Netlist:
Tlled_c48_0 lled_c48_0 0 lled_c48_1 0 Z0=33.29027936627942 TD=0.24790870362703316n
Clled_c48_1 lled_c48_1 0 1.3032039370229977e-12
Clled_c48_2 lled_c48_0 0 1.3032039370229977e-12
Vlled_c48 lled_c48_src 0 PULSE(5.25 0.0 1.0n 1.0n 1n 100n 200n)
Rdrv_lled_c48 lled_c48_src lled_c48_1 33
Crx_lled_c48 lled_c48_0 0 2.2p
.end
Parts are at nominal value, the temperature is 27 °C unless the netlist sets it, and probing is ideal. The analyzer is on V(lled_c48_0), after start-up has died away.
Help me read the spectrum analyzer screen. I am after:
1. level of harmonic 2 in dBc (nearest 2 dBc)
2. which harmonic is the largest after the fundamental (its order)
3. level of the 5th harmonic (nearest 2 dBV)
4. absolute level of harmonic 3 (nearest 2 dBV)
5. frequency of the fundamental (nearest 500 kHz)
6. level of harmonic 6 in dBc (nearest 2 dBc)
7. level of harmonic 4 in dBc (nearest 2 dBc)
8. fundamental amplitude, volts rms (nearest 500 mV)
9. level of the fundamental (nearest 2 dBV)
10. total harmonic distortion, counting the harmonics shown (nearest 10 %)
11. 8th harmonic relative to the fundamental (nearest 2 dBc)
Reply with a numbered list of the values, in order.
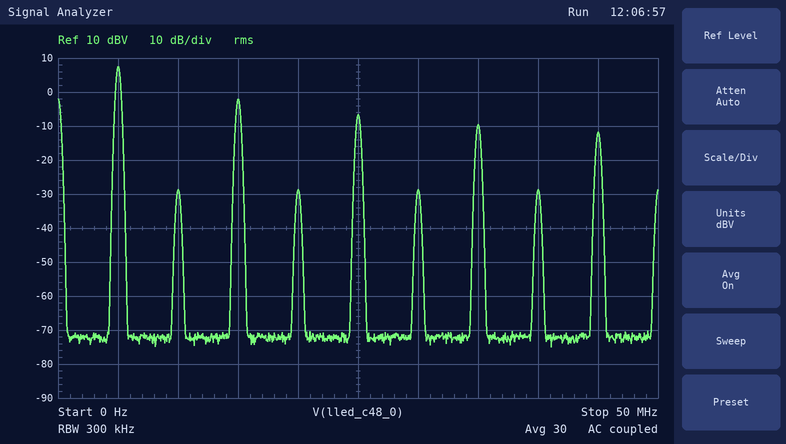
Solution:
1. -36 dBc
2. 3
3. -6 dBV
4. -2 dBV
5. 5.0 MHz
6. -36 dBc
7. -36 dBc
8. 2.5 V
9. 8 dBV
10. 40 %
11. -36 dBc
